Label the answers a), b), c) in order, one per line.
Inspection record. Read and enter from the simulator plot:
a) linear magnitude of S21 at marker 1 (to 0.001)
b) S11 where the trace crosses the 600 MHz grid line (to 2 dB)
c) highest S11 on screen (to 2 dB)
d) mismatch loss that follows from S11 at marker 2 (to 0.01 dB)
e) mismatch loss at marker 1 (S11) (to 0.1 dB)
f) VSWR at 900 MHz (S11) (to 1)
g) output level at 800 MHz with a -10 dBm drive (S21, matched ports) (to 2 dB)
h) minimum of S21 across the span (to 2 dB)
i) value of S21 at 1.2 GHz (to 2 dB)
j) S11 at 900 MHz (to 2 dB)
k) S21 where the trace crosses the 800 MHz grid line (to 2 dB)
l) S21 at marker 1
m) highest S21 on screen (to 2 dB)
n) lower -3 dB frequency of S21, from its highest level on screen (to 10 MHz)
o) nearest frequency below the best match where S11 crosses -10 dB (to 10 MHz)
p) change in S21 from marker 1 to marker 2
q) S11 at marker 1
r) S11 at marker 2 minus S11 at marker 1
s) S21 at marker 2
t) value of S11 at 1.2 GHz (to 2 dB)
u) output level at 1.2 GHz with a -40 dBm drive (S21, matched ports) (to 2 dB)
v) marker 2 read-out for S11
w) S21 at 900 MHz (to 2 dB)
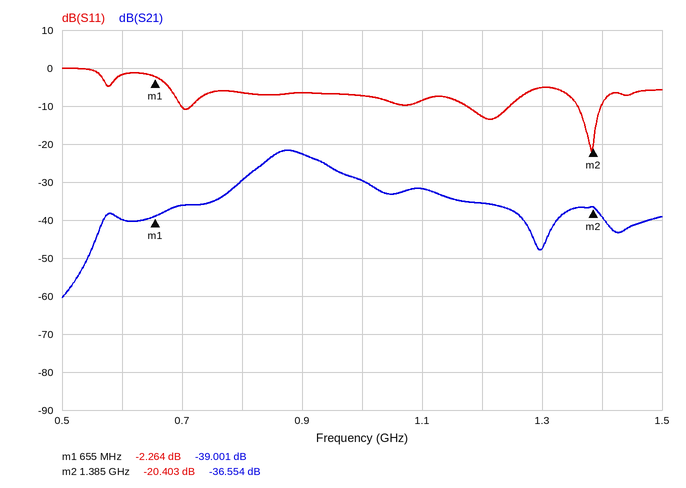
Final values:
a) 0.011
b) -2 dB
c) 0 dB
d) 0.04 dB
e) 3.9 dB
f) 3
g) -40 dBm
h) -60 dB
i) -36 dB
j) -6 dB
k) -30 dB
l) -39.001 dB
m) -22 dB
n) 840 MHz
o) 1.36 GHz
p) 2.447 dB
q) -2.264 dB
r) -18.139 dB
s) -36.554 dB
t) -12 dB
u) -76 dBm
v) -20.403 dB
w) -22 dB
